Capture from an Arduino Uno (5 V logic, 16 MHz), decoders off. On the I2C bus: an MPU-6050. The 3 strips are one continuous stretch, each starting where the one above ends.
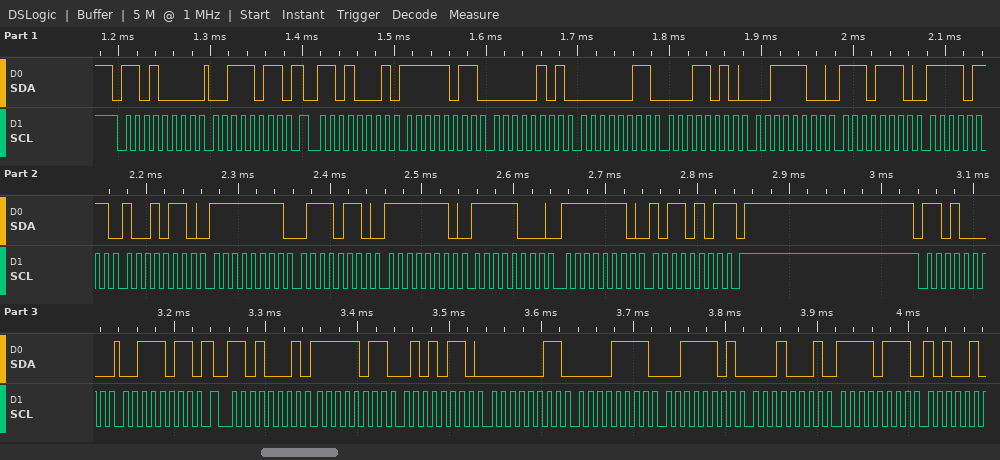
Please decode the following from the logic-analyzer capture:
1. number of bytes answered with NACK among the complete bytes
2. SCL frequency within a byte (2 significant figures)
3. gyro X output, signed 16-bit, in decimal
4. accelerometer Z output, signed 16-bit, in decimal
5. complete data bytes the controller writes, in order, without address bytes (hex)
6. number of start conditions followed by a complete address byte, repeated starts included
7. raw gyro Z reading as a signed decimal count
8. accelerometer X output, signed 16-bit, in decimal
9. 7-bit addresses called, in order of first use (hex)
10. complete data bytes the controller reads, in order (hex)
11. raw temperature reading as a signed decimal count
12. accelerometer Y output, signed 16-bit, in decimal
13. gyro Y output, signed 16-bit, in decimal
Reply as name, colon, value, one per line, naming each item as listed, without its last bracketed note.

number of bytes answered with NACK among the complete bytes: 1
SCL frequency within a byte: 100 kHz
gyro X output, signed 16-bit, in decimal: -138
accelerometer Z output, signed 16-bit, in decimal: 15598
complete data bytes the controller writes, in order, without address bytes: 3B 3B
number of start conditions followed by a complete address byte, repeated starts included: 4
raw gyro Z reading as a signed decimal count: -331
accelerometer X output, signed 16-bit, in decimal: -1275
7-bit addresses called, in order of first use: 0x68
complete data bytes the controller reads, in order: FB 05 03 1A 3C EE F7 96 FF 76 FE F8 FE B5 FB 56 03 0F 3D 11 F7
raw temperature reading as a signed decimal count: -2154
accelerometer Y output, signed 16-bit, in decimal: 794
gyro Y output, signed 16-bit, in decimal: -264
